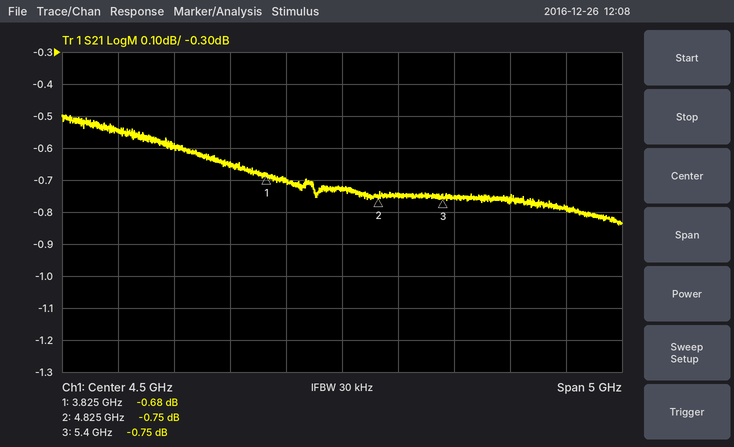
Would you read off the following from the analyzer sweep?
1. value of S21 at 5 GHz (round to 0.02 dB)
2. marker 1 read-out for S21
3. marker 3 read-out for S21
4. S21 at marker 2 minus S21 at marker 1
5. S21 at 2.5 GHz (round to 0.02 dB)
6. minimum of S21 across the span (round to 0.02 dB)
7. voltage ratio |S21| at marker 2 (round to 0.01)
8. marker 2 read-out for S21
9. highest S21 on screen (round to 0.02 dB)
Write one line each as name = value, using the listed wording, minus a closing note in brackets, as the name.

value of S21 at 5 GHz = -0.74 dB
marker 1 read-out for S21 = -0.68 dB
marker 3 read-out for S21 = -0.75 dB
S21 at marker 2 minus S21 at marker 1 = -0.07 dB
S21 at 2.5 GHz = -0.54 dB
minimum of S21 across the span = -0.84 dB
voltage ratio |S21| at marker 2 = 0.92
marker 2 read-out for S21 = -0.75 dB
highest S21 on screen = -0.50 dB
